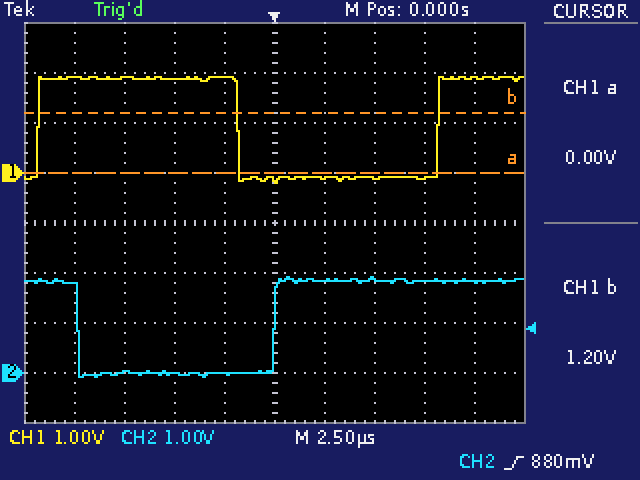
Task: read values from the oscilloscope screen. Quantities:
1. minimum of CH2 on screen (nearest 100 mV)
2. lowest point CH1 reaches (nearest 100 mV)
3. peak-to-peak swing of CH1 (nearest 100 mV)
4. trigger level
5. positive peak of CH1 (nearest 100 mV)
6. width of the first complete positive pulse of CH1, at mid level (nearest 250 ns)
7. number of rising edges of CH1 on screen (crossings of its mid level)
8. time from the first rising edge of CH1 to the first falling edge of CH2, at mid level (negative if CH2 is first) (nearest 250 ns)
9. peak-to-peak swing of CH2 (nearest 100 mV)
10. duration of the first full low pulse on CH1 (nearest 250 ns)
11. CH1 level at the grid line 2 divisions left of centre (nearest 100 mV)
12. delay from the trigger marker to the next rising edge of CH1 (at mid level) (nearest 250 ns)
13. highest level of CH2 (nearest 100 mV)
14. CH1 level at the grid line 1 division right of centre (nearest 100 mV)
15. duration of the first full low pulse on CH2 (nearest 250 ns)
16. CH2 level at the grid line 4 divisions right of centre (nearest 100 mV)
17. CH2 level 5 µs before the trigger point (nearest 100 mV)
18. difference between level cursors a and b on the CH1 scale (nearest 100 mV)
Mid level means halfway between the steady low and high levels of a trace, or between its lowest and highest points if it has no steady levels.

-100 mV
-200 mV
2.1 V
880 mV
1.9 V
10.00 µs
2
+2.00 µs
2.0 V
10.00 µs
1.9 V
8.25 µs
1.9 V
-100 mV
9.75 µs
1.8 V
0.0 V
1.2 V
